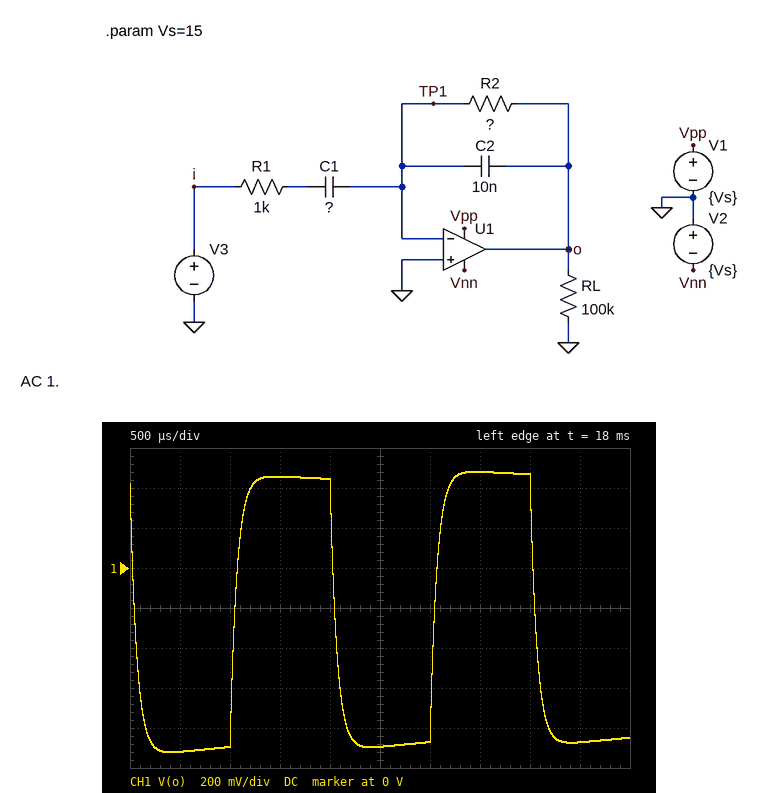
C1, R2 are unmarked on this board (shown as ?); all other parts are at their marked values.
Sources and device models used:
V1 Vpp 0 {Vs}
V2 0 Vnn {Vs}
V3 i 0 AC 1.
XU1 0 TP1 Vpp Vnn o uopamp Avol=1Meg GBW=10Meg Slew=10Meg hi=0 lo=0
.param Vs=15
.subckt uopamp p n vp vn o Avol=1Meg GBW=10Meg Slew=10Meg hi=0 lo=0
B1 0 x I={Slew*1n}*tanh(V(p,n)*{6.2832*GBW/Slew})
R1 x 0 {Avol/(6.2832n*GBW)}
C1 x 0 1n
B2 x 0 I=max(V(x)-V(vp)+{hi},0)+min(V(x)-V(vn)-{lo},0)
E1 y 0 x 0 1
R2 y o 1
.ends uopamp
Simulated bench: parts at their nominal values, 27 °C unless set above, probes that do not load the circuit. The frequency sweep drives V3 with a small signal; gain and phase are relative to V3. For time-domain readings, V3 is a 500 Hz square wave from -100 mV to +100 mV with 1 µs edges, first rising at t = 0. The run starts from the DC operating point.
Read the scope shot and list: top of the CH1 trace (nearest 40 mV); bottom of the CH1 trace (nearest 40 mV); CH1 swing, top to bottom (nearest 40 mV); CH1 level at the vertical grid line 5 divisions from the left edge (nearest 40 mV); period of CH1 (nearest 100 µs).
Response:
480 mV
-920 mV
1.40 V
-880 mV
2.0 ms
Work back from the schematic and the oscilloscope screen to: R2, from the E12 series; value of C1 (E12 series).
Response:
6.8 kΩ
18 µF
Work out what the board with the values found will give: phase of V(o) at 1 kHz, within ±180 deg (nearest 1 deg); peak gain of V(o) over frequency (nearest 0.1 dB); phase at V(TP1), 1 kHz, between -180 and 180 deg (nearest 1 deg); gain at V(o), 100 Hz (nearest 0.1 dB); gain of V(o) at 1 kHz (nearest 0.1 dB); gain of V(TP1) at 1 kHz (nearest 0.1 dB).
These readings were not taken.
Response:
157 deg
16.6 dB
67 deg
16.6 dB
15.9 dB
-64.1 dB
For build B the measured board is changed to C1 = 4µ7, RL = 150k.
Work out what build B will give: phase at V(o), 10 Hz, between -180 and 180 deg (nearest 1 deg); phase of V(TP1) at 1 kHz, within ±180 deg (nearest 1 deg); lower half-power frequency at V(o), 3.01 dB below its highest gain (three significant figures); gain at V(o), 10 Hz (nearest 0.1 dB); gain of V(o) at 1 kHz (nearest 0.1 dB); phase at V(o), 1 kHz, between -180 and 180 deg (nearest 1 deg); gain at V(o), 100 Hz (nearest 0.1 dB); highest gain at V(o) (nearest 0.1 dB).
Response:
-107 deg
68 deg
32.9 Hz
5.7 dB
15.9 dB
159 deg
16.2 dB
16.5 dB
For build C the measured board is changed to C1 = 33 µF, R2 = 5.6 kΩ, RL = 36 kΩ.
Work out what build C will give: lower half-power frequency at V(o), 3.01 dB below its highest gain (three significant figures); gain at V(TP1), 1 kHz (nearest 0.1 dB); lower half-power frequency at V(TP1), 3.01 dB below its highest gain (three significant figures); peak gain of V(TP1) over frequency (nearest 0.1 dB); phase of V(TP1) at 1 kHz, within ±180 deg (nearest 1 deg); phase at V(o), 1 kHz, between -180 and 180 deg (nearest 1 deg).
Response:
4.81 Hz
-65.5 dB
2.84 kHz
-56.0 dB
70 deg
161 deg
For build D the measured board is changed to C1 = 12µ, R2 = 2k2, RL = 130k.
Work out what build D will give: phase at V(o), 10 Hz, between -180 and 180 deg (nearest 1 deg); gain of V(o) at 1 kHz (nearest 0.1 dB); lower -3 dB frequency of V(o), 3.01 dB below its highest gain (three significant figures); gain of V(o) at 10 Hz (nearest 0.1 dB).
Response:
-127 deg
6.8 dB
13.2 Hz
2.4 dB
